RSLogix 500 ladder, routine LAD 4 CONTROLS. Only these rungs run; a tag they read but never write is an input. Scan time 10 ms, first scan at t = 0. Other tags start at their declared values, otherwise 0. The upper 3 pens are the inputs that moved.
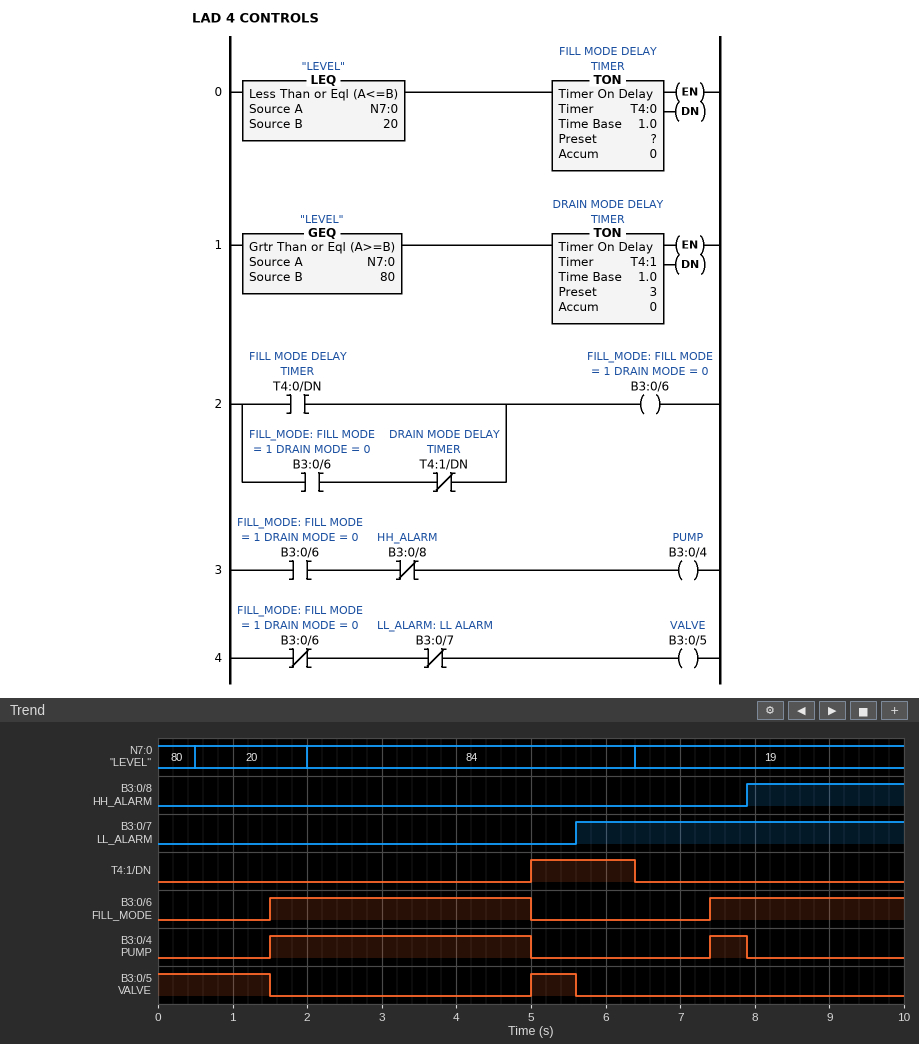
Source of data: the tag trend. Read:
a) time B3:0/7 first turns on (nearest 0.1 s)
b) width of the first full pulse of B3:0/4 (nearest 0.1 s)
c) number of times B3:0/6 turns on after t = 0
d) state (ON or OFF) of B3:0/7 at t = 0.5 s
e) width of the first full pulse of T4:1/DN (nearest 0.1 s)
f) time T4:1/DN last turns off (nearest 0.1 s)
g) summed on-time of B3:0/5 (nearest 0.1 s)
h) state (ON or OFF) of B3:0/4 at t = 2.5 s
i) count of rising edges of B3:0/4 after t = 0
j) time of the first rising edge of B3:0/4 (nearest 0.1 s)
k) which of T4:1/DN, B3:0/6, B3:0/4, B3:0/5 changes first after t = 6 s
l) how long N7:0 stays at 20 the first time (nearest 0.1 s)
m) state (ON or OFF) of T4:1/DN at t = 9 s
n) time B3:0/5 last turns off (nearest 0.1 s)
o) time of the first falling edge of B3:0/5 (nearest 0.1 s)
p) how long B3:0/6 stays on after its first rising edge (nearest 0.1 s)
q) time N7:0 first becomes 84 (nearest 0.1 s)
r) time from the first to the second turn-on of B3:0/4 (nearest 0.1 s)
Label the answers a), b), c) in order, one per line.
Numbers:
a) 5.6 s
b) 3.5 s
c) 2
d) OFF
e) 1.4 s
f) 6.4 s
g) 2.1 s
h) ON
i) 2
j) 1.5 s
k) T4:1/DN
l) 1.5 s
m) OFF
n) 5.6 s
o) 1.5 s
p) 3.5 s
q) 2.0 s
r) 5.9 s
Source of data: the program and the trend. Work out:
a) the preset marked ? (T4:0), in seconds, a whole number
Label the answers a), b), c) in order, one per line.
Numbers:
a) 1 s
